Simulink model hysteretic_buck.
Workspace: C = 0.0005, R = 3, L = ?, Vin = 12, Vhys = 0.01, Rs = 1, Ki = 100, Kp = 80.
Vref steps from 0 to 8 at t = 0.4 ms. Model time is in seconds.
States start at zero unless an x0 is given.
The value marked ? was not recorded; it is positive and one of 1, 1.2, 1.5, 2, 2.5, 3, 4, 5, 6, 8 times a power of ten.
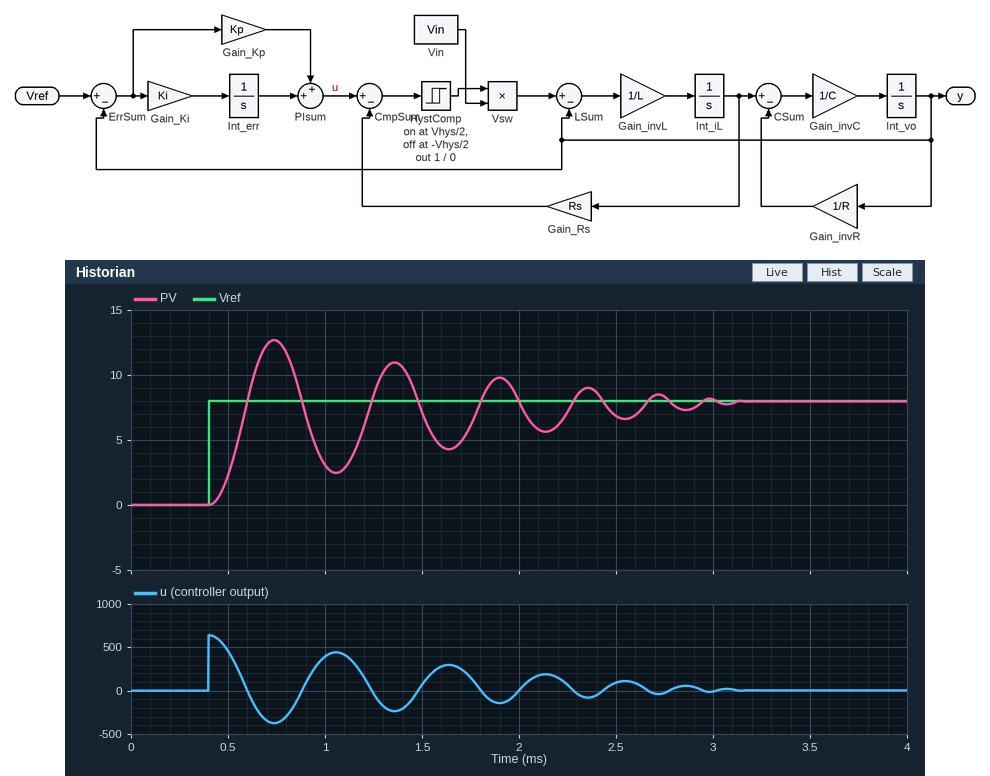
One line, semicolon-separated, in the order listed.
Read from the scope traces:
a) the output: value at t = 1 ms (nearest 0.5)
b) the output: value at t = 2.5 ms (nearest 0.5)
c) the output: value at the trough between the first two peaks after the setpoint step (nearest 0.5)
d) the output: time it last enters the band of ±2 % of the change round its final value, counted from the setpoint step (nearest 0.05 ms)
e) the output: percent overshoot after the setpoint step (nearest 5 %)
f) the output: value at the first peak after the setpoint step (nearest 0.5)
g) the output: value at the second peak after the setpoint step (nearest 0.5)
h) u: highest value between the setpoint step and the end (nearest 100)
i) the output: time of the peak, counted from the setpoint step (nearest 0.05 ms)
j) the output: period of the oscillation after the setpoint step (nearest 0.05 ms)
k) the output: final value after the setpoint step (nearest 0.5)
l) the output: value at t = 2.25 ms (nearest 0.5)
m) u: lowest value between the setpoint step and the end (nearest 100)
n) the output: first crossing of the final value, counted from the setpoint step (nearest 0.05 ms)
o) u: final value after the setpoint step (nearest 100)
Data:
3.0; 7.0; 2.5; 2.70 ms; 60 %; 12.5; 11.0; 600; 0.35 ms; 0.60 ms; 8.0; 7.0; -400; 0.20 ms; 0
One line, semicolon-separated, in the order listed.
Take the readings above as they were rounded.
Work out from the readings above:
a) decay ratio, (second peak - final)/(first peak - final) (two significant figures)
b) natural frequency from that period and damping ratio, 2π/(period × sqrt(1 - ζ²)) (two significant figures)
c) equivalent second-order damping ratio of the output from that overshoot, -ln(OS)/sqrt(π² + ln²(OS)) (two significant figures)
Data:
0.67; 11 rad/ms; 0.16
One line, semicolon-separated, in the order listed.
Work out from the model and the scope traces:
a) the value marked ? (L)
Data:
5e-05
